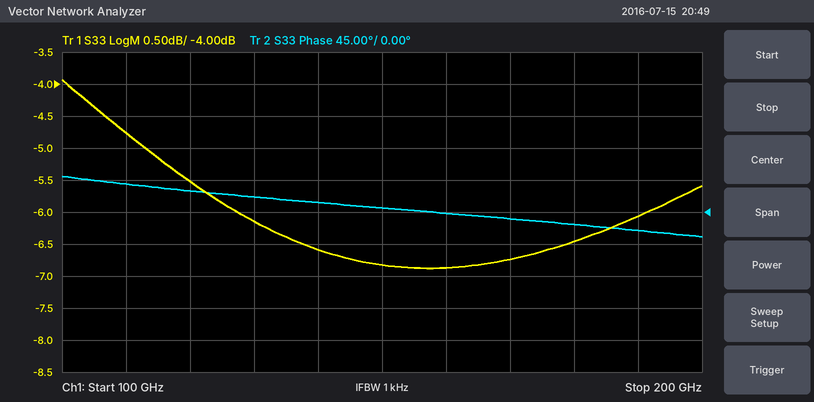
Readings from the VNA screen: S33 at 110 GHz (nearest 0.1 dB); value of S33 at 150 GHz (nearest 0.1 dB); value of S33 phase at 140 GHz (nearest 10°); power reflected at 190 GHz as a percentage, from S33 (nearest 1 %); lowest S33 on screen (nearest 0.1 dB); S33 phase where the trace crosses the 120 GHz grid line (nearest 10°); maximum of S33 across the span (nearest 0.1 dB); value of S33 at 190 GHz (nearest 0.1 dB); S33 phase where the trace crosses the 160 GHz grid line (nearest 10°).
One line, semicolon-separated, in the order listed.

-4.8 dB; -6.8 dB; 10°; 25 %; -6.9 dB; 30°; -3.9 dB; -6.1 dB; 0°
